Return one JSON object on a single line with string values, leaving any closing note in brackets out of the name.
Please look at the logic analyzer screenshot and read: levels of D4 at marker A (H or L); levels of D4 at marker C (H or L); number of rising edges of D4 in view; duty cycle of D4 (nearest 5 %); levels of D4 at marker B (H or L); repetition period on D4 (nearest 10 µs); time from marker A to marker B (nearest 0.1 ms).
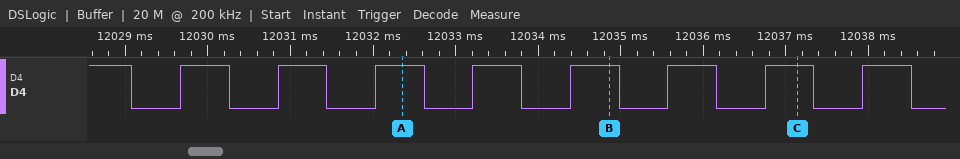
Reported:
{"levels of D4 at marker A": "D4=H", "levels of D4 at marker C": "D4=H", "number of rising edges of D4 in view": "8", "duty cycle of D4": "50 %", "levels of D4 at marker B": "D4=H", "repetition period on D4": "1180 µs", "time from marker A to marker B": "2.5 ms"}
